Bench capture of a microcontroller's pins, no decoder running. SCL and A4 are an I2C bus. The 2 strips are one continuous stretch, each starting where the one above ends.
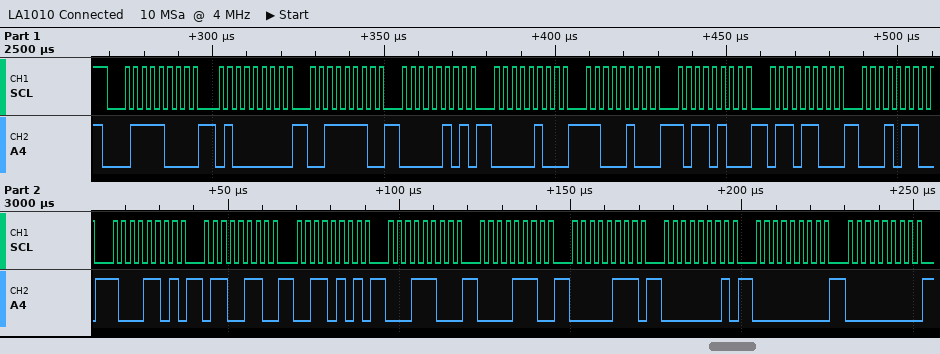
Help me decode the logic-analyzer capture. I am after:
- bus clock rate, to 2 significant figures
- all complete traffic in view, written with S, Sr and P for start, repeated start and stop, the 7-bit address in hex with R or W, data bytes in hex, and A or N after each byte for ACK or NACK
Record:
400 kHz
S 3CW A 40 A 3E A 05 A 04 A C4 A B4 A 6C A 16 A 8D A 66 A 35 A 1C A 0E A 07 A 01 A 00 A 00 A
